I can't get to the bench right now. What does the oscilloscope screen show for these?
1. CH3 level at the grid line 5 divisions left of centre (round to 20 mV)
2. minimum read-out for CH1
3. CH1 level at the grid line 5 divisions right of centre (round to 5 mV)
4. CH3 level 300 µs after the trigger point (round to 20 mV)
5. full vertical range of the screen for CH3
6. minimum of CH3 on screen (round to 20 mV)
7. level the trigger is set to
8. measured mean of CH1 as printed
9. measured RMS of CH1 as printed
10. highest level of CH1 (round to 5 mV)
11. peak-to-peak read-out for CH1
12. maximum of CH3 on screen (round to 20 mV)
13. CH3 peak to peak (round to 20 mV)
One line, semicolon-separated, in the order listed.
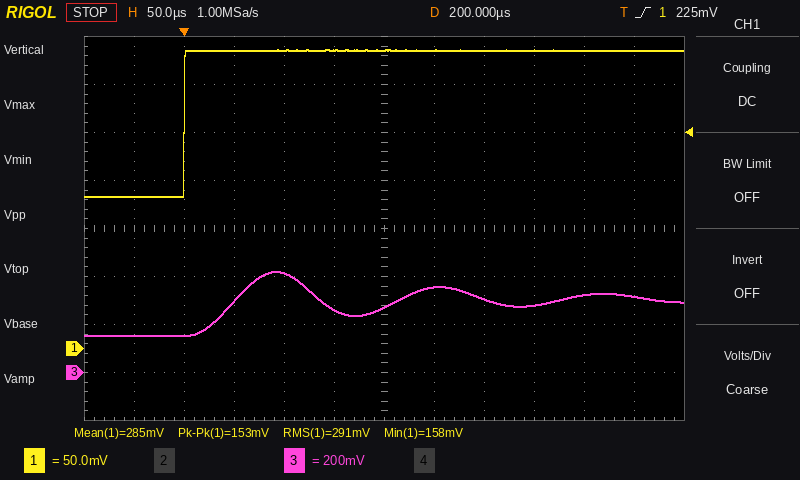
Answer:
160 mV; 158 mV; 310 mV; 300 mV; 1.6 V; 160 mV; 225 mV; 285 mV; 291 mV; 310 mV; 153 mV; 420 mV; 260 mV
